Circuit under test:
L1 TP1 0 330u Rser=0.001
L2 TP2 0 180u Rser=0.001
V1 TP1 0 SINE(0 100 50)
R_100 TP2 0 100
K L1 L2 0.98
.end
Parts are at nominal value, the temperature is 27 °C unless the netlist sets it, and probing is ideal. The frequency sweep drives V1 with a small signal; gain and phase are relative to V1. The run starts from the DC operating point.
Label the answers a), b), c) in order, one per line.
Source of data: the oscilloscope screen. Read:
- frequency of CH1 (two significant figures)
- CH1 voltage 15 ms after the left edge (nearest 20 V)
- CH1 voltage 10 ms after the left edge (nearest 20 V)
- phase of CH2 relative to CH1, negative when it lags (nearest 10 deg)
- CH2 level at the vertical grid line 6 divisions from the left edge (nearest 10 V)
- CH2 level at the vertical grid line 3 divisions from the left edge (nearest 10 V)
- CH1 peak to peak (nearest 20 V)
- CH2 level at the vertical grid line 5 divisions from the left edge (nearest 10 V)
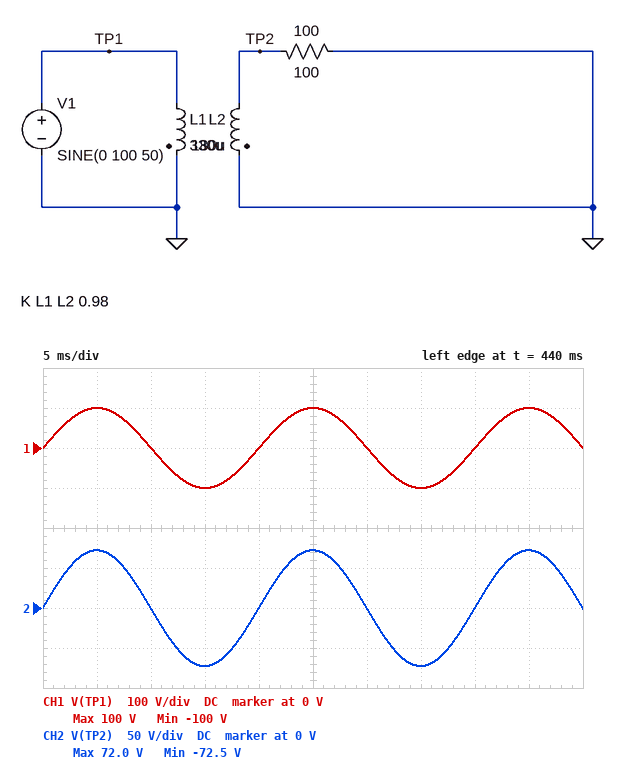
a) 50 Hz
b) -100 V
c) 0 V
d) 0 deg
e) 0 V
f) -70 V
g) 200 V
h) 70 V
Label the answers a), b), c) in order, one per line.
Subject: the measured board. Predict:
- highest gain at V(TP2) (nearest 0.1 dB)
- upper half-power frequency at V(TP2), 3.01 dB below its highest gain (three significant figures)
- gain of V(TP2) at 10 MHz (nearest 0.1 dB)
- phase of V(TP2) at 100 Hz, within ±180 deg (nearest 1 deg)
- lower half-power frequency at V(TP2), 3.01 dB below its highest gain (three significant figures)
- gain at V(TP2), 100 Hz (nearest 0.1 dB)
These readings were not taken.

a) -2.8 dB
b) 2.23 MHz
c) -16.0 dB
d) 0 deg
e) 482 mHz
f) -2.8 dB
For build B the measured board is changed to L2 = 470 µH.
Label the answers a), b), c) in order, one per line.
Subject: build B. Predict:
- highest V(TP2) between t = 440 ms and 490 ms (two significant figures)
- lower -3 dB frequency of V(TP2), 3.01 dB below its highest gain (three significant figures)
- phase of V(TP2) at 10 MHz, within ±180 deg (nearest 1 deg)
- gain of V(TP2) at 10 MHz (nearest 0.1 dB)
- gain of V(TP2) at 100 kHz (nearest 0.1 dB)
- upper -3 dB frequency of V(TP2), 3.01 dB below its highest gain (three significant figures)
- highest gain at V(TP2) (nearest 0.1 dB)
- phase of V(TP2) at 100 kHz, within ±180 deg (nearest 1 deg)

a) 120 V
b) 482 mHz
c) -85 deg
d) -20.0 dB
e) 1.3 dB
f) 855 kHz
g) 1.4 dB
h) -7 deg
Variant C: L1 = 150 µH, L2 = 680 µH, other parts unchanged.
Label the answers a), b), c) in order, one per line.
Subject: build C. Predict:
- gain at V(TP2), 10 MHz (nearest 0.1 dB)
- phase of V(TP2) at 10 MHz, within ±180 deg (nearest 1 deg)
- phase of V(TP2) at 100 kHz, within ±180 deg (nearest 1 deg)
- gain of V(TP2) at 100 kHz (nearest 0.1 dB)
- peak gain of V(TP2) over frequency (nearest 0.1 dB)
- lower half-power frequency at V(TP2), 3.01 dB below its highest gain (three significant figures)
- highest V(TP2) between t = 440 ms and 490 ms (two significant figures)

a) -18.2 dB
b) -87 deg
c) -10 deg
d) 6.3 dB
e) 6.4 dB
f) 1.06 Hz
g) 210 V
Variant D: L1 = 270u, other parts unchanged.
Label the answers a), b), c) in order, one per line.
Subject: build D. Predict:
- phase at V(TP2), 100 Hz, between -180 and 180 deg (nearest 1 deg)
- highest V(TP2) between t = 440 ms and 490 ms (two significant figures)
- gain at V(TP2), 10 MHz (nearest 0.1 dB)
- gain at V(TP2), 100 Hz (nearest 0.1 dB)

a) 0 deg
b) 80 V
c) -15.2 dB
d) -1.9 dB
